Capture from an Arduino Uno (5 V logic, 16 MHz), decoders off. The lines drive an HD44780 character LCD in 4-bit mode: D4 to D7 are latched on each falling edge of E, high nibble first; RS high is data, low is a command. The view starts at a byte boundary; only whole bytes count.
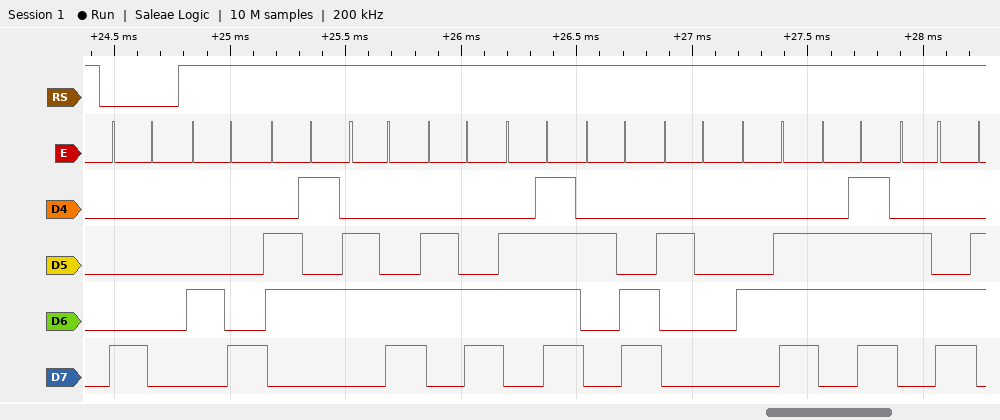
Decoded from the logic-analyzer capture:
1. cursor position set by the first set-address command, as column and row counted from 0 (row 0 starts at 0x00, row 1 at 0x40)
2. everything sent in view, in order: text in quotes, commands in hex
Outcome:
column 0, row 0
0x80 "Hello, Nol"
